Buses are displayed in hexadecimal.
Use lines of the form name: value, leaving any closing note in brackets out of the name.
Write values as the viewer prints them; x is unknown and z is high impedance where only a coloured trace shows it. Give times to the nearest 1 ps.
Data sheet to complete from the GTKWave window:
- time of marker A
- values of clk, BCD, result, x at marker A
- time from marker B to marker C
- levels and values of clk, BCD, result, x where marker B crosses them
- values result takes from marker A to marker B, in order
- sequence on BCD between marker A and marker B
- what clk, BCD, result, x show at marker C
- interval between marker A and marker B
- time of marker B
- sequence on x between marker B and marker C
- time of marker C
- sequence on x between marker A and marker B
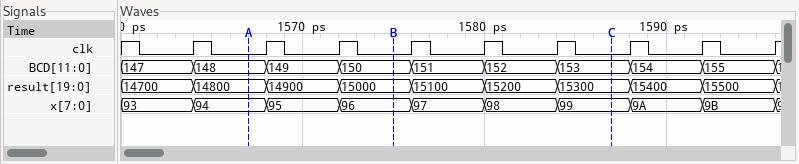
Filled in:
time of marker A: 1567 ps
values of clk, BCD, result, x at marker A: clk=0, BCD=148, result=14800, x=94
time from marker B to marker C: 12 ps
levels and values of clk, BCD, result, x where marker B crosses them: clk=0, BCD=150, result=15000, x=96
values result takes from marker A to marker B, in order: 14800, 14900, 15000
sequence on BCD between marker A and marker B: 148, 149, 150
what clk, BCD, result, x show at marker C: clk=0, BCD=153, result=15300, x=99
interval between marker A and marker B: 8 ps
time of marker B: 1575 ps
sequence on x between marker B and marker C: 96, 97, 98, 99
time of marker C: 1587 ps
sequence on x between marker A and marker B: 94, 95, 96
